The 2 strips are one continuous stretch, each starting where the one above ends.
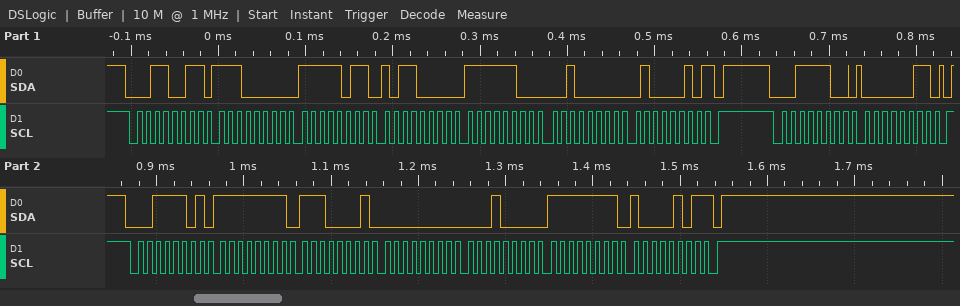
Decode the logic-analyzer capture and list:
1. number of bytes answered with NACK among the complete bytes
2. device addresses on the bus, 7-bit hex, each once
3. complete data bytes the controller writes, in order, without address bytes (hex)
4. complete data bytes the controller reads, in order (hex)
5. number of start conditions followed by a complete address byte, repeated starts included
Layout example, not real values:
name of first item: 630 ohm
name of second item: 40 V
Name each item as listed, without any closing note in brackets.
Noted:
number of bytes answered with NACK among the complete bytes: 2
device addresses on the bus, 7-bit hex, each once: 0x19 0x1E
complete data bytes the controller writes, in order, without address bytes: 03
complete data bytes the controller reads, in order: E0 FB B0 FC 20 42 FF E1 00 10 FF 85
number of start conditions followed by a complete address byte, repeated starts included: 3
